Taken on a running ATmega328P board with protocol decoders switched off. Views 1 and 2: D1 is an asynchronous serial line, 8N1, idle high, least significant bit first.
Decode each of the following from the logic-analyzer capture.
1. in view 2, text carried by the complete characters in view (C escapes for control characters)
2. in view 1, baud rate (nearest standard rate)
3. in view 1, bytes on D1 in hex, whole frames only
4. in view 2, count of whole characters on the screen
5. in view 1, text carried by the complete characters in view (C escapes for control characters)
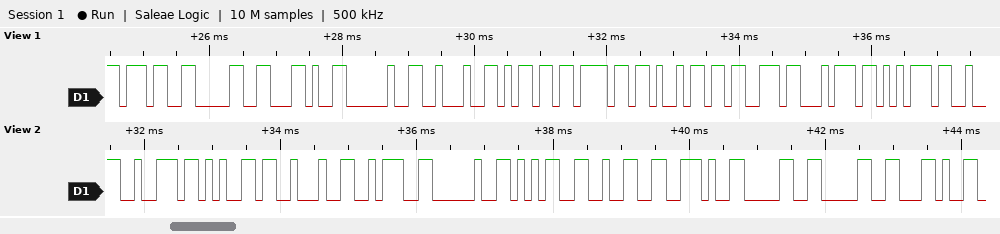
"re\": 52.00,"
9600 baud
37 30 2C 20 22 6D 6F 69 73 74 75
11
"70, \"moistu"
